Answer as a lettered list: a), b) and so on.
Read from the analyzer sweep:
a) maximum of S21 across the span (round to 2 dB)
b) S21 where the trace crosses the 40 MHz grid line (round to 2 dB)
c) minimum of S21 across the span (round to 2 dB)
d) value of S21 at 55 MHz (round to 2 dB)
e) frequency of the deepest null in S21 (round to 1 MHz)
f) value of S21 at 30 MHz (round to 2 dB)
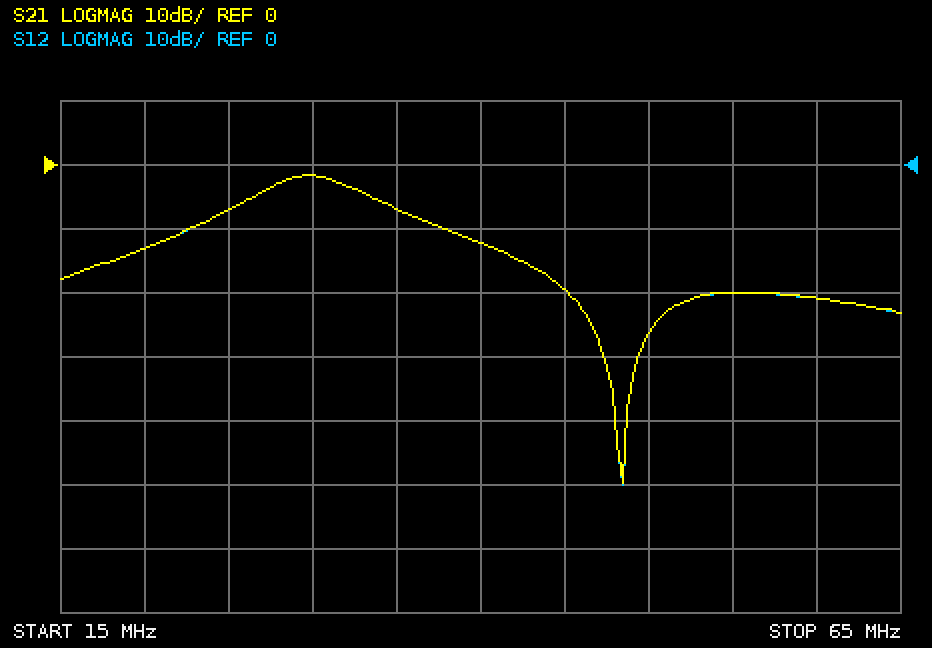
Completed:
a) -2 dB
b) -12 dB
c) -50 dB
d) -20 dB
e) 48 MHz
f) -2 dB
